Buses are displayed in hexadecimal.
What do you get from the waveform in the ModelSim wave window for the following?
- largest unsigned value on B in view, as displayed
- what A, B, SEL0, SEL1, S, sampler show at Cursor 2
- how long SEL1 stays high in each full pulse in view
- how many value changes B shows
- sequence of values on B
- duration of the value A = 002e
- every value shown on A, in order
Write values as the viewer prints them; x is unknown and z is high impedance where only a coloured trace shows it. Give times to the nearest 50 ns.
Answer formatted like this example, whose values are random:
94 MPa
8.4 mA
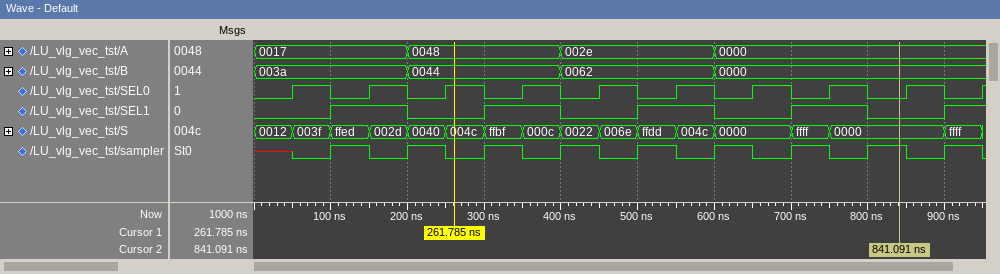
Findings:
0062
A=0000, B=0000, SEL0=0, SEL1=0, S=0000, sampler=1
100 ns, 100 ns, 100 ns, 100 ns
3
003a, 0044, 0062, 0000
200 ns
0017, 0048, 002e, 0000
